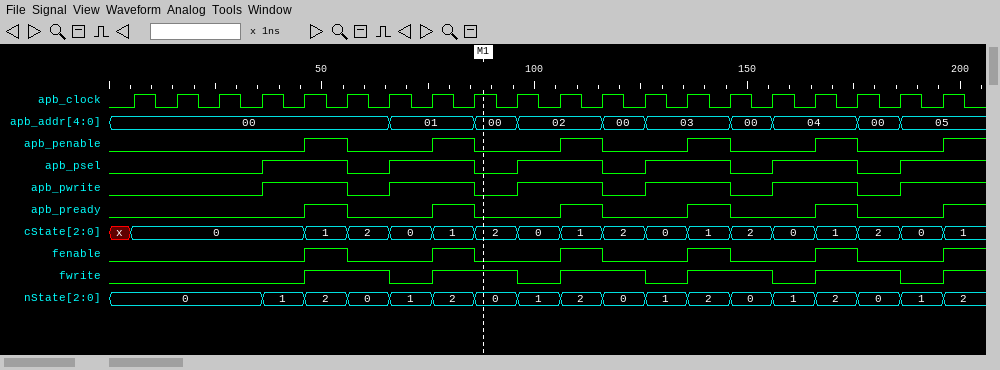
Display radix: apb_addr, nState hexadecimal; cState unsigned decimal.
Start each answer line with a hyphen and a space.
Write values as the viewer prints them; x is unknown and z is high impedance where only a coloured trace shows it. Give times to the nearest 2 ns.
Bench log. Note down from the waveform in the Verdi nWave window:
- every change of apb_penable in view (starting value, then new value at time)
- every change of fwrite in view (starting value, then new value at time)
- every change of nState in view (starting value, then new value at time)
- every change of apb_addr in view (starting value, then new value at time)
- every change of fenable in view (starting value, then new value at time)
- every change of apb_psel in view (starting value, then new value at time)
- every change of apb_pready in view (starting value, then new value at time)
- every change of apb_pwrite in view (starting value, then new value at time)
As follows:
- 0, 1 at 46 ns, 0 at 56 ns, 1 at 76 ns, 0 at 86 ns, 1 at 106 ns, 0 at 116 ns, 1 at 136 ns, 0 at 146 ns, 1 at 166 ns, 0 at 176 ns, 1 at 196 ns
- 0, 1 at 46 ns, 0 at 66 ns, 1 at 76 ns, 0 at 96 ns, 1 at 106 ns, 0 at 126 ns, 1 at 136 ns, 0 at 156 ns, 1 at 166 ns, 0 at 186 ns, 1 at 196 ns
- 0, 1 at 36 ns, 2 at 46 ns, 0 at 56 ns, 1 at 66 ns, 2 at 76 ns, 0 at 86 ns, 1 at 96 ns, 2 at 106 ns, 0 at 116 ns, 1 at 126 ns, 2 at 136 ns, 0 at 146 ns, 1 at 156 ns, 2 at 166 ns, 0 at 176 ns, 1 at 186 ns, 2 at 196 ns
- 00, 01 at 66 ns, 00 at 86 ns, 02 at 96 ns, 00 at 116 ns, 03 at 126 ns, 00 at 146 ns, 04 at 156 ns, 00 at 176 ns, 05 at 186 ns
- 0, 1 at 46 ns, 0 at 56 ns, 1 at 76 ns, 0 at 86 ns, 1 at 106 ns, 0 at 116 ns, 1 at 136 ns, 0 at 146 ns, 1 at 166 ns, 0 at 176 ns, 1 at 196 ns
- 0, 1 at 36 ns, 0 at 56 ns, 1 at 66 ns, 0 at 86 ns, 1 at 96 ns, 0 at 116 ns, 1 at 126 ns, 0 at 146 ns, 1 at 156 ns, 0 at 176 ns, 1 at 186 ns
- 0, 1 at 46 ns, 0 at 56 ns, 1 at 76 ns, 0 at 86 ns, 1 at 106 ns, 0 at 116 ns, 1 at 136 ns, 0 at 146 ns, 1 at 166 ns, 0 at 176 ns, 1 at 196 ns
- 0, 1 at 36 ns, 0 at 56 ns, 1 at 66 ns, 0 at 86 ns, 1 at 96 ns, 0 at 116 ns, 1 at 126 ns, 0 at 146 ns, 1 at 156 ns, 0 at 176 ns, 1 at 186 ns
